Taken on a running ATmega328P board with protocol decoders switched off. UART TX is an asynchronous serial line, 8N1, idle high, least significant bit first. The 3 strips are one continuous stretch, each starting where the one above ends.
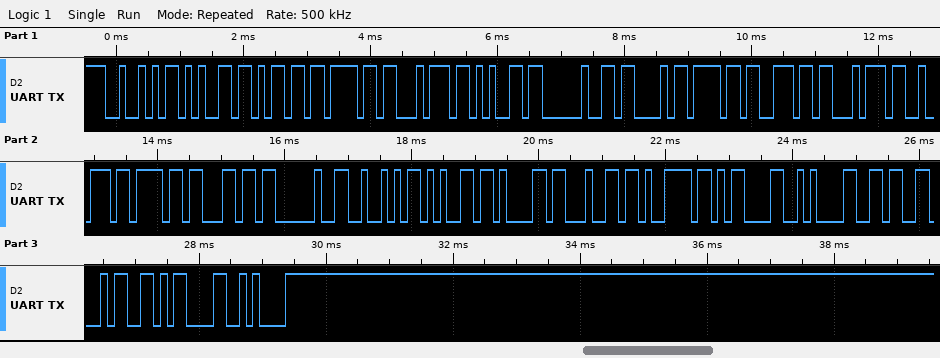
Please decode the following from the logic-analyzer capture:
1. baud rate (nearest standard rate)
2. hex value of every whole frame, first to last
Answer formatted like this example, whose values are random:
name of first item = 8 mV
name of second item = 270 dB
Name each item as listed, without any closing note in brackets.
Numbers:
baud rate = 9600 baud
hex value of every whole frame, first to last = 52 65 6D 6F 74 65 20 43 6F 6E 74 72 6F 6C 20 52 65 61 64 79 0D 0A 36 34 0D 0A
